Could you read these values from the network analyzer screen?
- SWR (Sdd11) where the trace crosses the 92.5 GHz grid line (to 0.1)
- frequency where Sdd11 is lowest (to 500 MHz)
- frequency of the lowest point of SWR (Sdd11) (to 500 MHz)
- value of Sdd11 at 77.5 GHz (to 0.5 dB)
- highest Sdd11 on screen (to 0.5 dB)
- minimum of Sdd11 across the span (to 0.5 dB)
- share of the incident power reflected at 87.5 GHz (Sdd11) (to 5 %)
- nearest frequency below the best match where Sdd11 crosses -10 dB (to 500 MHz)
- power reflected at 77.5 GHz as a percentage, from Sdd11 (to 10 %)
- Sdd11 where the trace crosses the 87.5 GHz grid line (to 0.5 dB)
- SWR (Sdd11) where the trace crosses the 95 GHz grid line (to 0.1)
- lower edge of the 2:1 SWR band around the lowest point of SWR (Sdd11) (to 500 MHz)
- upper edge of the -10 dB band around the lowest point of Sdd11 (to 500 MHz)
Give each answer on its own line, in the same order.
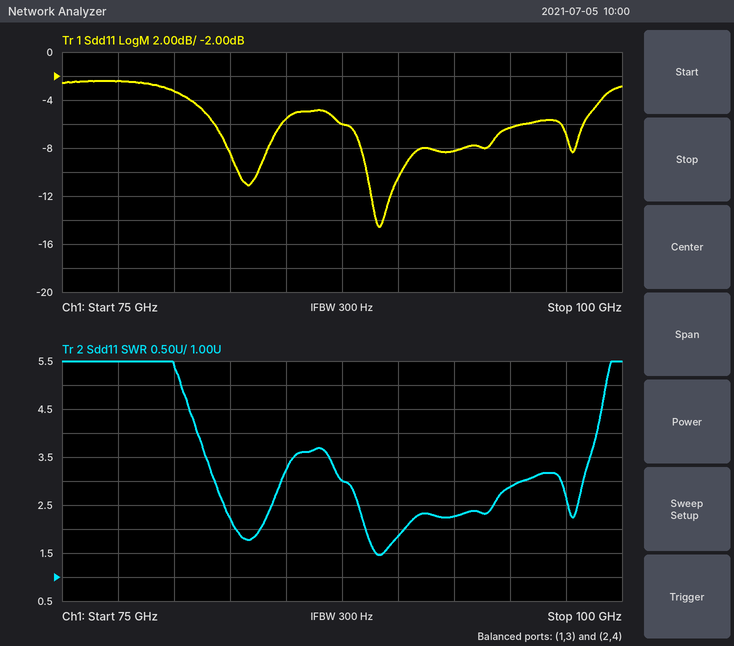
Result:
2.3
89.0 GHz
89.0 GHz
-2.5 dB
-2.5 dB
-14.5 dB
25 %
88.5 GHz
60 %
-6.0 dB
2.9
88.5 GHz
90.0 GHz
